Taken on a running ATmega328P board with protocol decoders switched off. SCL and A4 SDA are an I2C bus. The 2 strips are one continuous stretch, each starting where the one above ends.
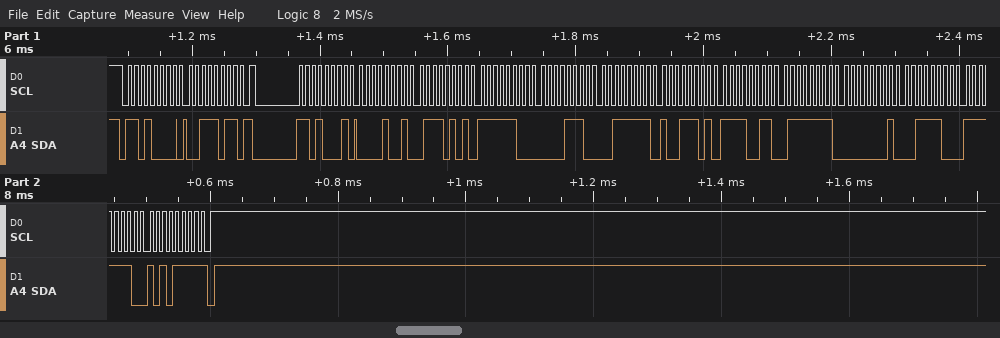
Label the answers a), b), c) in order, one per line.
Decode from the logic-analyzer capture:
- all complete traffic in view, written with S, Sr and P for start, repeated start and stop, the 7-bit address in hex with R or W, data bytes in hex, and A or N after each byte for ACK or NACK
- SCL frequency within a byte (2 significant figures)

a) S 68W A 3B A Sr 68R A 09 A 75 A FC A 0E A 3F A 9D A F3 A 7F A 01 A 3C A FE A AF N P
b) 100 kHz
